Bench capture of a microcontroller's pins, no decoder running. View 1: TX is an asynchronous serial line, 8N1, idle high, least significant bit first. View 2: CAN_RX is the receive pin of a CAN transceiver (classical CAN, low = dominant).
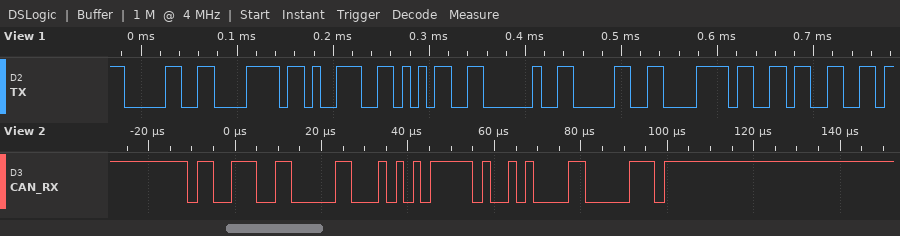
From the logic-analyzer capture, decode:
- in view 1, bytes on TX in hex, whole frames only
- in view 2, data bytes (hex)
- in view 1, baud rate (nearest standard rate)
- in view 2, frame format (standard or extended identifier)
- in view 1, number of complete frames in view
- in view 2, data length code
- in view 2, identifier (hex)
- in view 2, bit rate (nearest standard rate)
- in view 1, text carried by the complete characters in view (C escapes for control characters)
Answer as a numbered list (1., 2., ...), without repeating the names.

1. 0x30 0x78 0x39 0x35 0x20 0x30 0x78 0x36
2. 2A FC
3. 115200 baud
4. standard
5. 8
6. 2
7. 0x673
8. 500 kbit/s
9. "0x95 0x6"
